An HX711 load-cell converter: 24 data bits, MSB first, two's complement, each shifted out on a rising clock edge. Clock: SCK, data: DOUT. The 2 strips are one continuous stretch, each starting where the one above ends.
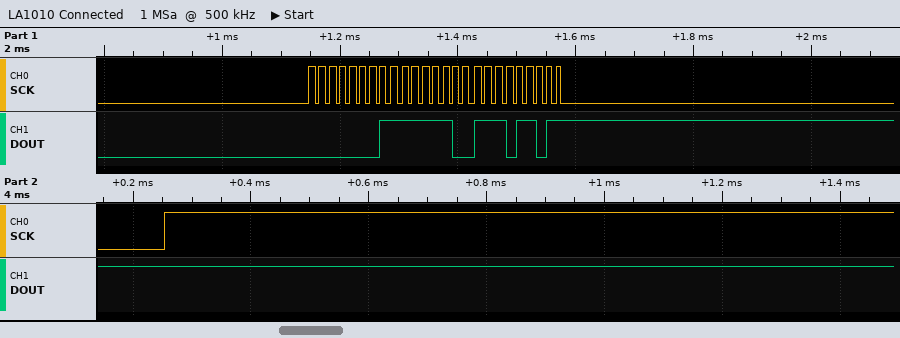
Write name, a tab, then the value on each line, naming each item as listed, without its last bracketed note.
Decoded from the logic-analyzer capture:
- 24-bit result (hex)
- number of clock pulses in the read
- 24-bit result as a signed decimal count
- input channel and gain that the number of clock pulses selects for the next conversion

24-bit result	0x01FCED
number of clock pulses in the read	26
24-bit result as a signed decimal count	130285
input channel and gain that the number of clock pulses selects for the next conversion	channel B, gain 32
